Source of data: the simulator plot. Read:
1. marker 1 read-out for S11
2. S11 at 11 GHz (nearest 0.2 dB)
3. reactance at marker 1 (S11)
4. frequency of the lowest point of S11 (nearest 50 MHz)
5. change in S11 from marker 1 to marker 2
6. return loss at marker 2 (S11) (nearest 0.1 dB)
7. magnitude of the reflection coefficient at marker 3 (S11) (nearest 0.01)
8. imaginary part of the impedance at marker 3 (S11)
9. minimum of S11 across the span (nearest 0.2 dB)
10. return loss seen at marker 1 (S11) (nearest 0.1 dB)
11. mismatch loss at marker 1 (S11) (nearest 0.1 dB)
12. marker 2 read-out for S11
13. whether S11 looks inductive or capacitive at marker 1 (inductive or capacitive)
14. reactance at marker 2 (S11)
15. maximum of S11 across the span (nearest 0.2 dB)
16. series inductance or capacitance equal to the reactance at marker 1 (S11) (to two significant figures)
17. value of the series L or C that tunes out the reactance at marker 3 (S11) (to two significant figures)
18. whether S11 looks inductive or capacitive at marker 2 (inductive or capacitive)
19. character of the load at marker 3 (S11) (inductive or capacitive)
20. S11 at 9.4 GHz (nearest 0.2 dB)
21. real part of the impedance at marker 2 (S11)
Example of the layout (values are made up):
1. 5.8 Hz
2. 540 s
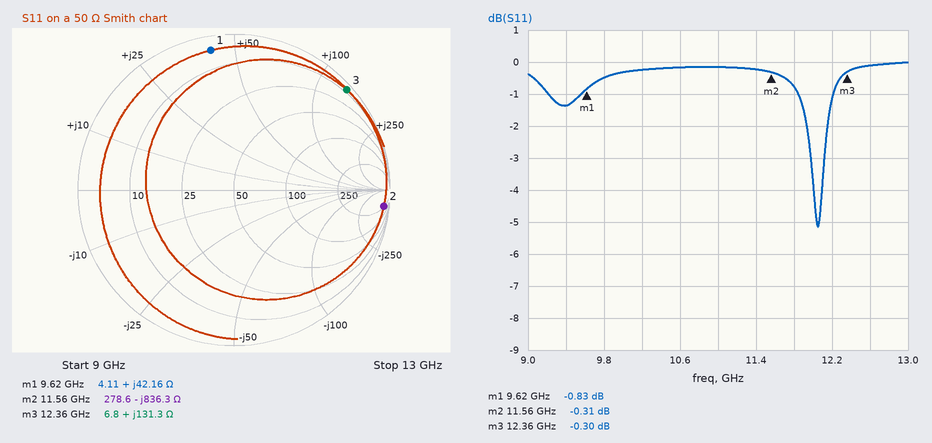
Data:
1. -0.83 dB
2. -0.2 dB
3. +42.16 Ω
4. 12.05 GHz
5. 0.52 dB
6. 0.3 dB
7. 0.97
8. +131.3 Ω
9. -5.2 dB
10. 0.8 dB
11. 7.6 dB
12. -0.31 dB
13. inductive
14. -836.3 Ω
15. 0.0 dB
16. 700 pH
17. 98 fF
18. capacitive
19. inductive
20. -1.4 dB
21. 278.6 Ω
